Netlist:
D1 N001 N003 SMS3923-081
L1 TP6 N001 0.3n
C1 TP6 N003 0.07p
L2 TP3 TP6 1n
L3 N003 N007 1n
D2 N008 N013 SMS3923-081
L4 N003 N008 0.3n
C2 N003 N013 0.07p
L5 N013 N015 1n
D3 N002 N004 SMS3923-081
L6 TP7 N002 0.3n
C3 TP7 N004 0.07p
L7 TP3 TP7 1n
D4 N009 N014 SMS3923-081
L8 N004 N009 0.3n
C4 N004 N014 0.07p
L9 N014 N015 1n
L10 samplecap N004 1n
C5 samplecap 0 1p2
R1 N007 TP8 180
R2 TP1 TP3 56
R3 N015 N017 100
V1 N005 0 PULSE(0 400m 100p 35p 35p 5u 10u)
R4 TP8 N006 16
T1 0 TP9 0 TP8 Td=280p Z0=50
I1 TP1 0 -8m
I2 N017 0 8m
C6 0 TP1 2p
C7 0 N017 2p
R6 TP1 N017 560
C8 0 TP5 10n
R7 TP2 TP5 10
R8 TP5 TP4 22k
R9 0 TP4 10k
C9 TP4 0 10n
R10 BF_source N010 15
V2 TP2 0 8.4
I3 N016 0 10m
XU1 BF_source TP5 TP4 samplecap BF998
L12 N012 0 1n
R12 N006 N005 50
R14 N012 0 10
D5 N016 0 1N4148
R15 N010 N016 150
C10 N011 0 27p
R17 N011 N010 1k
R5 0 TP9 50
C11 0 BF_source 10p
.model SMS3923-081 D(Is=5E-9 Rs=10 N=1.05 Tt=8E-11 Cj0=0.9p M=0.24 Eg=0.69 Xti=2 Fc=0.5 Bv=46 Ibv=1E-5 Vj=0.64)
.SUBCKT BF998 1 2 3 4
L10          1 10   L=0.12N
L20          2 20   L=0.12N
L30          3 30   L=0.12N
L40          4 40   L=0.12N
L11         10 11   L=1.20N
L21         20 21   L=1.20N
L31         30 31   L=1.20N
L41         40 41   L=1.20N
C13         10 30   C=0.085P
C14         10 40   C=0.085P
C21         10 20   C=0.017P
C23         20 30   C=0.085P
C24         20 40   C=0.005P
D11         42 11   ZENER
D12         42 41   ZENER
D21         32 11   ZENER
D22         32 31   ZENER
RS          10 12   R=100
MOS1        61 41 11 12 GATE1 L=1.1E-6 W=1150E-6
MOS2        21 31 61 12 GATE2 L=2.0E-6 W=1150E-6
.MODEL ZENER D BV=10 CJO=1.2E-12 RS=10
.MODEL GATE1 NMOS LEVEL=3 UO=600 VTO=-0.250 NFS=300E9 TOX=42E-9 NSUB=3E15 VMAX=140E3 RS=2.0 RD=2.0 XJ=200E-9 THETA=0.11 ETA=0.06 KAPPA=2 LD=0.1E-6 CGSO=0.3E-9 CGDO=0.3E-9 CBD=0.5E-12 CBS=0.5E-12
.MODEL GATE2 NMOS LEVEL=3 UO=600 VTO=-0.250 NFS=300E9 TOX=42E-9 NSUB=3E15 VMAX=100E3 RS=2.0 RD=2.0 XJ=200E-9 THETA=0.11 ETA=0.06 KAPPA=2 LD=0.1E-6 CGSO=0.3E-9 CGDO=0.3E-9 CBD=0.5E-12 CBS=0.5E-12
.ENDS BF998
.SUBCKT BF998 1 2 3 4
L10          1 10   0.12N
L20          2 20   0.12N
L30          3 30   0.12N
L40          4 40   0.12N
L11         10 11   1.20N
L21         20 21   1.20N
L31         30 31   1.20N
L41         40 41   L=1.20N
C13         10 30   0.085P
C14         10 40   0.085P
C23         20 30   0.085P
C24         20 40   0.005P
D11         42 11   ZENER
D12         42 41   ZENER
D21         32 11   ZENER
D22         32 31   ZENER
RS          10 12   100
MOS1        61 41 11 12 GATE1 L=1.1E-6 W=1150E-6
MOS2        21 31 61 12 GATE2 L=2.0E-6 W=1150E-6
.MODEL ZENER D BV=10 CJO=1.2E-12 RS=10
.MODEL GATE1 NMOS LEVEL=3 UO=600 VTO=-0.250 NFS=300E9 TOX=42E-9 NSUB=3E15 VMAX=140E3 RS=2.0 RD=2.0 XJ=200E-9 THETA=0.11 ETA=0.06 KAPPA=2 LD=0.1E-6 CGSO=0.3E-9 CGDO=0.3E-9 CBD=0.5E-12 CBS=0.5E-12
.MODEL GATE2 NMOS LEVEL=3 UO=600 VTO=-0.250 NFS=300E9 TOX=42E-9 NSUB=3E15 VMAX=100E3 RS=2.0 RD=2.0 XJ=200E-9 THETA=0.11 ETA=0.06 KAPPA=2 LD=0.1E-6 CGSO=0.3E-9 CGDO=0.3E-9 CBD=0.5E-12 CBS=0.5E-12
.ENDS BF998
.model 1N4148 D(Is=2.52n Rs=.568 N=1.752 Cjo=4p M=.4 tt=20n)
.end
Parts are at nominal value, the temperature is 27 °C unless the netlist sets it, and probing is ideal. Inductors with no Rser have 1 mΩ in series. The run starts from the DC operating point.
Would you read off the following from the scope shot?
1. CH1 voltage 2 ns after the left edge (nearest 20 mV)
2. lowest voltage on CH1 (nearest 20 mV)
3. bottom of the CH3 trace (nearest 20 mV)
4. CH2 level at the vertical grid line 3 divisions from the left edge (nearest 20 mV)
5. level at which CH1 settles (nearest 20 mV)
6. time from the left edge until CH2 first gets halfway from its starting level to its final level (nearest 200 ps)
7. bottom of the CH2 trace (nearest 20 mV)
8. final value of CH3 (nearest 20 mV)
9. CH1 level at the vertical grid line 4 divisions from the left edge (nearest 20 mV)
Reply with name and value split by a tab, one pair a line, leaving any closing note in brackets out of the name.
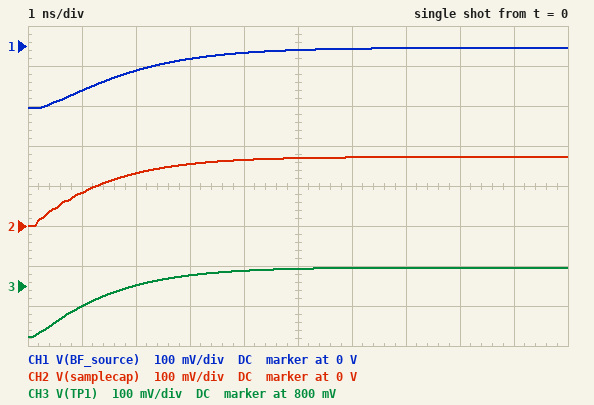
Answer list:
CH1 voltage 2 ns after the left edge	-60 mV
lowest voltage on CH1	-160 mV
bottom of the CH3 trace	680 mV
CH2 level at the vertical grid line 3 divisions from the left edge	160 mV
level at which CH1 settles	0 V
time from the left edge until CH2 first gets halfway from its starting level to its final level	1.0 ns
bottom of the CH2 trace	0 V
final value of CH3	840 mV
CH1 level at the vertical grid line 4 divisions from the left edge	-20 mV
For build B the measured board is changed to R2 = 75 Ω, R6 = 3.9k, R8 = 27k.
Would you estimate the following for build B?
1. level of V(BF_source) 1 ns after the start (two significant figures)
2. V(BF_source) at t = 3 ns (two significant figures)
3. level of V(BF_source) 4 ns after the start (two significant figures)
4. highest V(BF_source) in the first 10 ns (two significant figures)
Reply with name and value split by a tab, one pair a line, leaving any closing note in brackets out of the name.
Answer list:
level of V(BF_source) 1 ns after the start	-140 mV
V(BF_source) at t = 3 ns	-65 mV
level of V(BF_source) 4 ns after the start	-50 mV
highest V(BF_source) in the first 10 ns	-37 mV
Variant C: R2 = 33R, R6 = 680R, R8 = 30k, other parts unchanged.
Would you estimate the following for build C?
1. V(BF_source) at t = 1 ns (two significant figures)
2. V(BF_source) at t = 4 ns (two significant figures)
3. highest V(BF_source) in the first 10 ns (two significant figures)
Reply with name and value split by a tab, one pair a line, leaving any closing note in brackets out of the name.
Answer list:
V(BF_source) at t = 1 ns	-160 mV
V(BF_source) at t = 4 ns	-65 mV
highest V(BF_source) in the first 10 ns	-52 mV
